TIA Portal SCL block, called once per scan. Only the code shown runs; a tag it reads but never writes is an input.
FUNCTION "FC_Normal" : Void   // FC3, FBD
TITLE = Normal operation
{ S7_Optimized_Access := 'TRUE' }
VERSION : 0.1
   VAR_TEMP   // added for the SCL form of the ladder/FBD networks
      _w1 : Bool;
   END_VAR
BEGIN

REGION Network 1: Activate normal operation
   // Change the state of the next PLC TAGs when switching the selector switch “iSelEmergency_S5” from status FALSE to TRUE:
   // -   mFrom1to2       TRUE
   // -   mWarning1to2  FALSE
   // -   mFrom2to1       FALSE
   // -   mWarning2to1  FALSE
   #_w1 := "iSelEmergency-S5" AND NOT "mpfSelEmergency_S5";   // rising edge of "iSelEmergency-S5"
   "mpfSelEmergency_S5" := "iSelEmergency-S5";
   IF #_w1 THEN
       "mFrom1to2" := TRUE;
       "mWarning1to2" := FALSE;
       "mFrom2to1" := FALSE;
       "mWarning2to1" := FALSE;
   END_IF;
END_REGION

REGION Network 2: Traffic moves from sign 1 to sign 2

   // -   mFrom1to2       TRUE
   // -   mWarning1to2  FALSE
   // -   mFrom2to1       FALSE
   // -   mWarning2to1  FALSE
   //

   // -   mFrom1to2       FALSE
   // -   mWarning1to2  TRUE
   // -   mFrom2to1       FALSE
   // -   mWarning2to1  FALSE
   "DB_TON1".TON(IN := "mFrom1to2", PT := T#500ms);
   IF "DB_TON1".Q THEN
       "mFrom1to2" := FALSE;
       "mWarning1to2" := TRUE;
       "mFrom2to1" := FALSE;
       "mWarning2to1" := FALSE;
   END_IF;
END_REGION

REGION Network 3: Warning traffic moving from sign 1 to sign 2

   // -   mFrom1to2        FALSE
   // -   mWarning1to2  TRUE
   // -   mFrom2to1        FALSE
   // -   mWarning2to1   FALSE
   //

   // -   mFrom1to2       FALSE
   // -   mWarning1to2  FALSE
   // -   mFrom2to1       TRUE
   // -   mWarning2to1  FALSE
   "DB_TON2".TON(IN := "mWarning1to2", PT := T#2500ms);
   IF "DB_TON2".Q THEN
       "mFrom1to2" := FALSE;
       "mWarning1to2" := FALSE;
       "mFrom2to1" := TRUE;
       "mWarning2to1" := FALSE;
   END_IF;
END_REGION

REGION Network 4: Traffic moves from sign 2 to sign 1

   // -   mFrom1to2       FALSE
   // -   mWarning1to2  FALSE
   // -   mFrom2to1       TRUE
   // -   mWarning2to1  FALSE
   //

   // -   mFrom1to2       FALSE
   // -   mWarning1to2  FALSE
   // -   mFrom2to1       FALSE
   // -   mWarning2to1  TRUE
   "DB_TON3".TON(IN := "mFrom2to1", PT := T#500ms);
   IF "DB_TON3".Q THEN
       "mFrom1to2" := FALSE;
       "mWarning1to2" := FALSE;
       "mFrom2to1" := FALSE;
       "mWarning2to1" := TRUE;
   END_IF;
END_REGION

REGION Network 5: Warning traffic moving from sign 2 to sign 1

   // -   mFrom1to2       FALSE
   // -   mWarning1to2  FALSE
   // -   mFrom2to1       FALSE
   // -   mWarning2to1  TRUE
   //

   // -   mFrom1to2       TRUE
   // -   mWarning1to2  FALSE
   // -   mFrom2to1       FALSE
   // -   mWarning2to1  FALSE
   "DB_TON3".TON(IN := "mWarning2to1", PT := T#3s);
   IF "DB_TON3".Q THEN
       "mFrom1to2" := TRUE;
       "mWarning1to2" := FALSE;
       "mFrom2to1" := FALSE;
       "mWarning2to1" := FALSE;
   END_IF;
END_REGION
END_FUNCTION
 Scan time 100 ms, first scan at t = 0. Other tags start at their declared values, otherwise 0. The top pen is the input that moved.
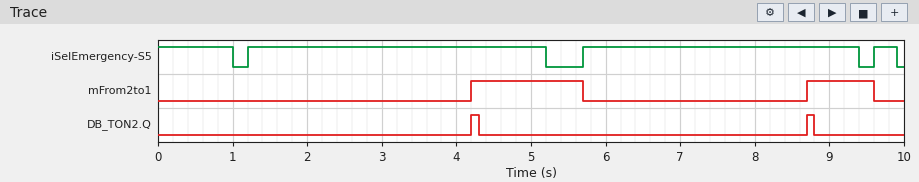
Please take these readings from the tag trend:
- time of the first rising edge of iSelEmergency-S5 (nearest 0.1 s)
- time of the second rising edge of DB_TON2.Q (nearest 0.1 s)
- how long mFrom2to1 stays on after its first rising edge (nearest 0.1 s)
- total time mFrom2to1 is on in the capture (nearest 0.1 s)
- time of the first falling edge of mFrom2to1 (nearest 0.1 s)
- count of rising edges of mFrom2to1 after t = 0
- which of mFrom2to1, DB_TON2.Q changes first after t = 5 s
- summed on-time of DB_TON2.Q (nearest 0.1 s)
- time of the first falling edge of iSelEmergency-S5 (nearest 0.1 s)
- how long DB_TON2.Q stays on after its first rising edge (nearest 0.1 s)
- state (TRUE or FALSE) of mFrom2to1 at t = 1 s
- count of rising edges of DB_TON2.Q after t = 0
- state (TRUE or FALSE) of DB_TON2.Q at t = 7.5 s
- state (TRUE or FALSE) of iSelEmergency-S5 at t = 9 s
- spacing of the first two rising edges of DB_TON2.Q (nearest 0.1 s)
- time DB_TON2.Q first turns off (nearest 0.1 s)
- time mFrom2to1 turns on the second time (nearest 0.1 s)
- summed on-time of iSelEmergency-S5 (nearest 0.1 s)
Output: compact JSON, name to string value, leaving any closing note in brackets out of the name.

{"time of the first rising edge of iSelEmergency-S5": "1.2 s", "time of the second rising edge of DB_TON2.Q": "8.7 s", "how long mFrom2to1 stays on after its first rising edge": "1.5 s", "total time mFrom2to1 is on in the capture": "2.4 s", "time of the first falling edge of mFrom2to1": "5.7 s", "count of rising edges of mFrom2to1 after t = 0": "2", "which of mFrom2to1, DB_TON2.Q changes first after t = 5 s": "mFrom2to1", "summed on-time of DB_TON2.Q": "0.2 s", "time of the first falling edge of iSelEmergency-S5": "1.0 s", "how long DB_TON2.Q stays on after its first rising edge": "0.1 s", "state (TRUE or FALSE) of mFrom2to1 at t = 1 s": "FALSE", "count of rising edges of DB_TON2.Q after t = 0": "2", "state (TRUE or FALSE) of DB_TON2.Q at t = 7.5 s": "FALSE", "state (TRUE or FALSE) of iSelEmergency-S5 at t = 9 s": "TRUE", "spacing of the first two rising edges of DB_TON2.Q": "4.5 s", "time DB_TON2.Q first turns off": "4.3 s", "time mFrom2to1 turns on the second time": "8.7 s", "summed on-time of iSelEmergency-S5": "9.0 s"}
